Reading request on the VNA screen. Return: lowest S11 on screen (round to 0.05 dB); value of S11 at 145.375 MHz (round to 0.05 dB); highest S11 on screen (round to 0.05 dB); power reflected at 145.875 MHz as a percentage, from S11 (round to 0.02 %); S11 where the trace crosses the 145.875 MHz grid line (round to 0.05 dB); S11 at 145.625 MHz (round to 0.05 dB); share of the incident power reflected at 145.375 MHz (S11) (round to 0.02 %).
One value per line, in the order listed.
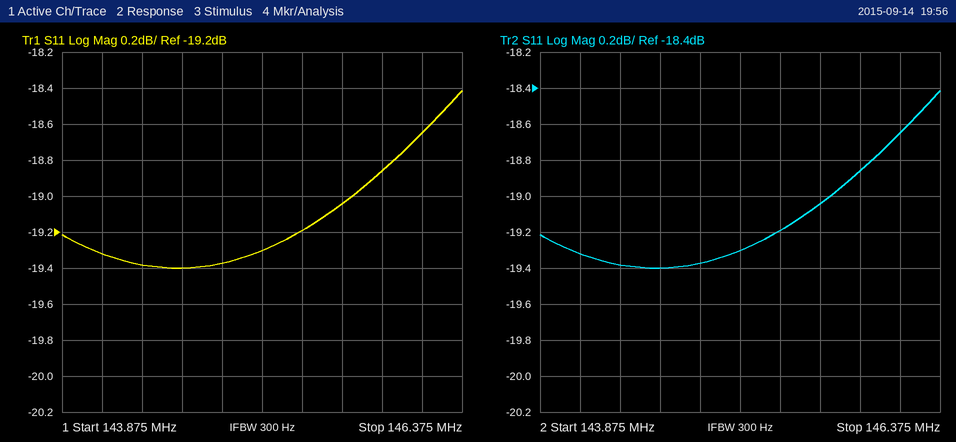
-19.40 dB
-19.20 dB
-18.40 dB
1.30 %
-18.85 dB
-19.05 dB
1.20 %
